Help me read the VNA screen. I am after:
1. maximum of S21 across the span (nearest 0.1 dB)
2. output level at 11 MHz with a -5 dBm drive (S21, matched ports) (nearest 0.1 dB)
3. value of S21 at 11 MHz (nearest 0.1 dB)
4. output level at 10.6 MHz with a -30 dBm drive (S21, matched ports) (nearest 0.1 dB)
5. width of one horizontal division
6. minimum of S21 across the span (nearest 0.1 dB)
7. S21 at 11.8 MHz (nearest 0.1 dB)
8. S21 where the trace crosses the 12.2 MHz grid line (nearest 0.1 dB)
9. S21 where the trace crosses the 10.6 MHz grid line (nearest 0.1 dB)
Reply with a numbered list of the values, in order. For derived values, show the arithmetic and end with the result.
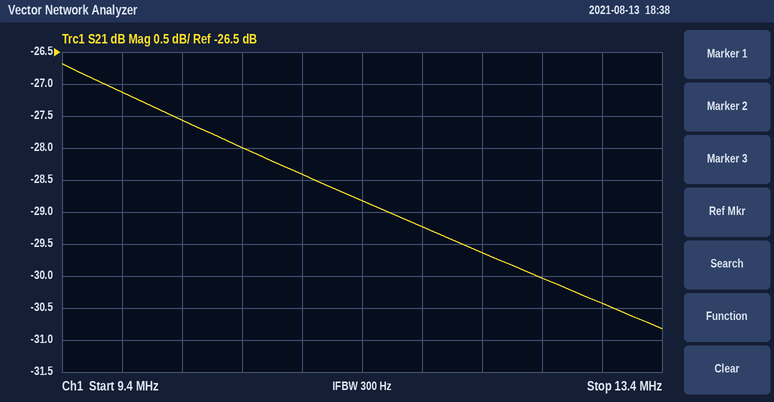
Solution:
1. -26.7 dB
2. -5 dBm + (-28.4 dB) = -33.4 dBm
3. -28.4 dB
4. -30 dBm + (-28.0 dB) = -58.0 dBm
5. 400 kHz
6. -30.8 dB
7. -29.2 dB
8. -29.6 dB
9. -28.0 dB
